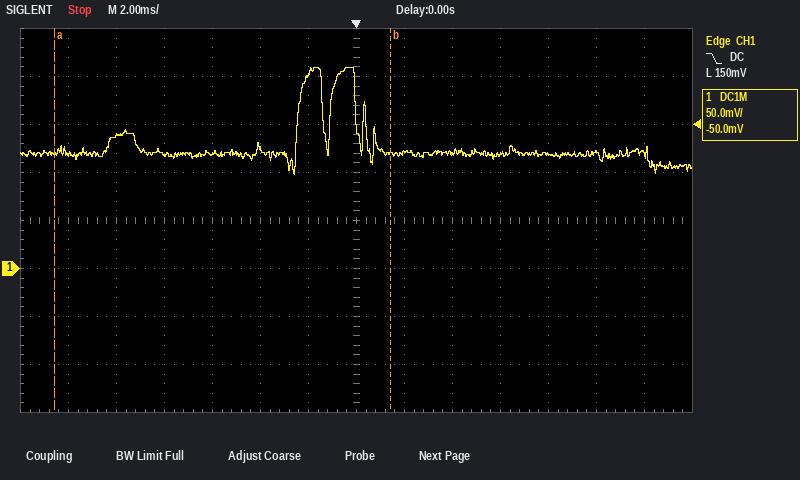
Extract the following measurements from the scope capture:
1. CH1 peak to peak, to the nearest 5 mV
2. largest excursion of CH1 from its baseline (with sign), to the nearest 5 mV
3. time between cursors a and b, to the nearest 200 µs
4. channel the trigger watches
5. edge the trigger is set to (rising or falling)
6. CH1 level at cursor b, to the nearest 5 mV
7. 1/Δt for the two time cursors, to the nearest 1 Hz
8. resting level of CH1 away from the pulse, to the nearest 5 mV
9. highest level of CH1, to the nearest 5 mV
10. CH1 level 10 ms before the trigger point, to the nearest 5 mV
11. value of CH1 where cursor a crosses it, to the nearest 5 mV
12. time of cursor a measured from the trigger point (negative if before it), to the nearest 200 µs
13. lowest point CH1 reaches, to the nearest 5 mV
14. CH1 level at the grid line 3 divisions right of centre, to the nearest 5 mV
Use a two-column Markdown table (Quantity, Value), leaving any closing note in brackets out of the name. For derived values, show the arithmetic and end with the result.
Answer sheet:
| Quantity | Value |
|---|---|
| CH1 peak to peak, to the nearest 5 mV | 210 mV − (100 mV) = 110 mV |
| largest excursion of CH1 from its baseline (with sign), to the nearest 5 mV | 210 mV − (120 mV) = +90 mV |
| time between cursors a and b, to the nearest 200 µs | 14.0 ms |
| channel the trigger watches | CH1 |
| edge the trigger is set to | falling |
| CH1 level at cursor b, to the nearest 5 mV | 120 mV |
| 1/Δt for the two time cursors, to the nearest 1 Hz | 1 / 14.0 ms ≈ 71 Hz |
| resting level of CH1 away from the pulse, to the nearest 5 mV | 120 mV |
| highest level of CH1, to the nearest 5 mV | 210 mV |
| CH1 level 10 ms before the trigger point, to the nearest 5 mV | 140 mV |
| value of CH1 where cursor a crosses it, to the nearest 5 mV | 120 mV |
| time of cursor a measured from the trigger point (negative if before it), to the nearest 200 µs | -12.6 ms |
| lowest point CH1 reaches, to the nearest 5 mV | 100 mV |
| CH1 level at the grid line 3 divisions right of centre, to the nearest 5 mV | 120 mV |
